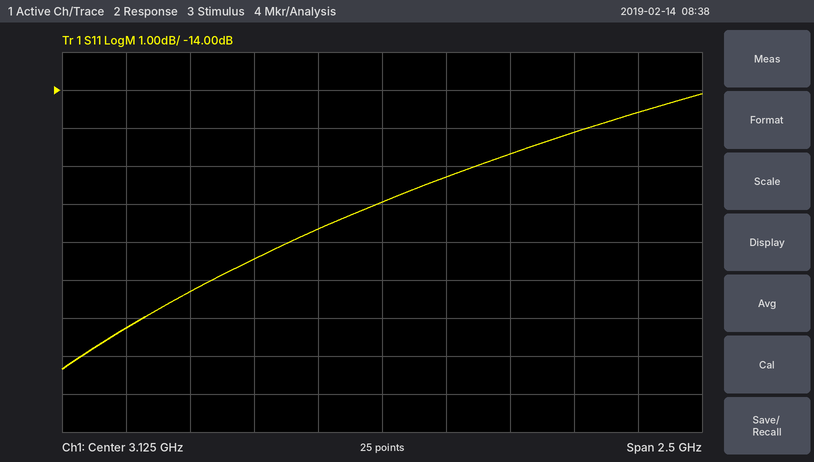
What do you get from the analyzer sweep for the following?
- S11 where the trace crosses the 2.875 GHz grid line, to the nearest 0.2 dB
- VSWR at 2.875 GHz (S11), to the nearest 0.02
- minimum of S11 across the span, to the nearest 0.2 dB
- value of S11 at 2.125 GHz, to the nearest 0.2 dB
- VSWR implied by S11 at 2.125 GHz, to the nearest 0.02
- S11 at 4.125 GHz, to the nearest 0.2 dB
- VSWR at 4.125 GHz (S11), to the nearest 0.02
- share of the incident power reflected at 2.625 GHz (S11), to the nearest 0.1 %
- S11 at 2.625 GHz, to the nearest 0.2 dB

-17.6 dB
1.30
-21.4 dB
-20.2 dB
1.22
-14.6 dB
1.46
1.4 %
-18.4 dB
